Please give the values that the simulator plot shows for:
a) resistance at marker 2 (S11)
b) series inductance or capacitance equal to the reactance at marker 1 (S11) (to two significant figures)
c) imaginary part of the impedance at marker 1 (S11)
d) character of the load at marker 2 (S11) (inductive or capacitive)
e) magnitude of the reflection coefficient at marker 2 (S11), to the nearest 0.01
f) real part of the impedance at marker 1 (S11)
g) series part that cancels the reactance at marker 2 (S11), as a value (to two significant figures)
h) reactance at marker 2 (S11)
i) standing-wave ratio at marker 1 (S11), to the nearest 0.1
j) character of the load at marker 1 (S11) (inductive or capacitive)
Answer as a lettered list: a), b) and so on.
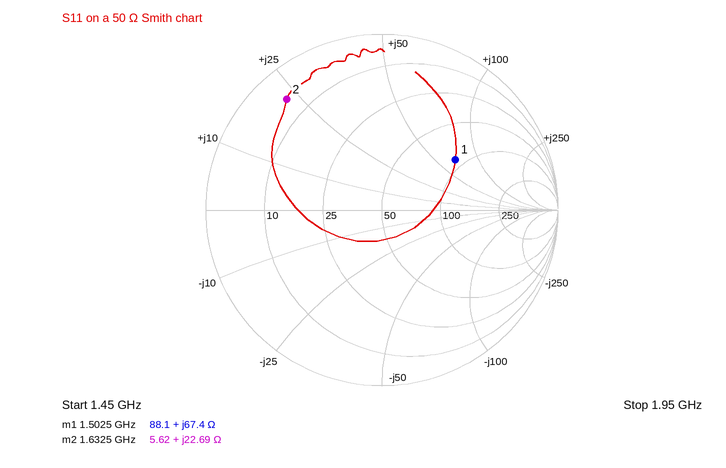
a) 5.62 Ω
b) 7.1 nH
c) +67.4 Ω
d) inductive
e) 0.83
f) 88.1 Ω
g) 4.3 pF
h) +22.69 Ω
i) 3.0
j) inductive
